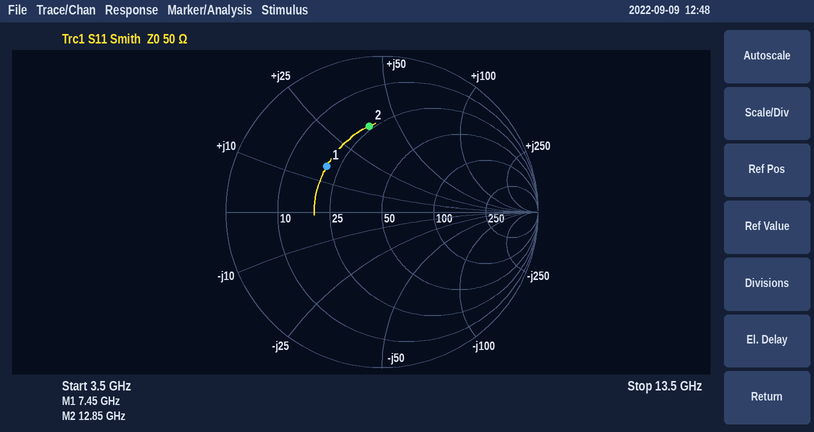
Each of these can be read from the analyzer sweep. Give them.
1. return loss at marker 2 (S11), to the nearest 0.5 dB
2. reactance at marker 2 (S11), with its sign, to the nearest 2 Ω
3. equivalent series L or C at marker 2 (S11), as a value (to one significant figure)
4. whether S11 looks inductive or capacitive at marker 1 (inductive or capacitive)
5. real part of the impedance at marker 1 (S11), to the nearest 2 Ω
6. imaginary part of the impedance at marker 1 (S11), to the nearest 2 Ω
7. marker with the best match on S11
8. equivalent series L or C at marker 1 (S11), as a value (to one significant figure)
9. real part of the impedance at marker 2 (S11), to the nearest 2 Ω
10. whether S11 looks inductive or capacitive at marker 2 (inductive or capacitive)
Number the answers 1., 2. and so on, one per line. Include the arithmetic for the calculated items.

1. 5.0 dB
2. +38 Ω
3. L = 38 Ω/(2π × 12.85 GHz) ≈ 471 pH, so 500 pH to one significant figure
4. inductive
5. 20 Ω
6. +16 Ω
7. marker 1
8. L = 16 Ω/(2π × 7.45 GHz) ≈ 342 pH, so 300 pH to one significant figure
9. 24 Ω
10. inductive
